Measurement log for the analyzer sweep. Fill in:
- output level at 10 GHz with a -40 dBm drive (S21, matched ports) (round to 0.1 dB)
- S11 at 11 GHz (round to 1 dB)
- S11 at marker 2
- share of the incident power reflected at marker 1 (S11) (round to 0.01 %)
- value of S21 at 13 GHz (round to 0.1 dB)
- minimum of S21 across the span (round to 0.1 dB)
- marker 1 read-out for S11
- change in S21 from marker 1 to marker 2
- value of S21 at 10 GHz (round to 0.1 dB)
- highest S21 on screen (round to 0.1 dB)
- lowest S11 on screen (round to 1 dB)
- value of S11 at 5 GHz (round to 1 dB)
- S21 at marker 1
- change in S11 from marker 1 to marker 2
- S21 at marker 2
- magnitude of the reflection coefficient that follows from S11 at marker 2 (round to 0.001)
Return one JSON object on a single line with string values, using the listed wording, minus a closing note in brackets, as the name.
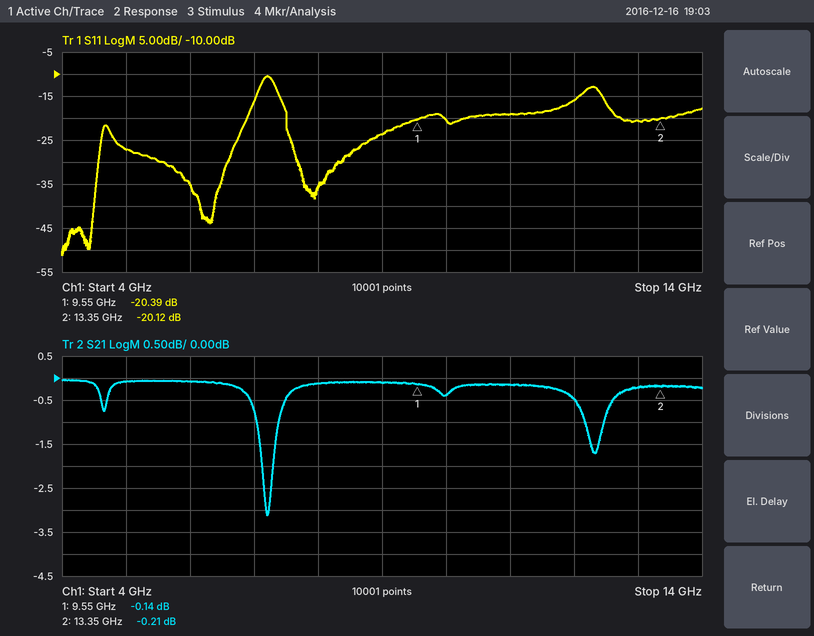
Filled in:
{"output level at 10 GHz with a -40 dBm drive (S21, matched ports)": "-40.4 dBm", "S11 at 11 GHz": "-19 dB", "S11 at marker 2": "-20.12 dB", "share of the incident power reflected at marker 1 (S11)": "0.91 %", "value of S21 at 13 GHz": "-0.2 dB", "minimum of S21 across the span": "-3.1 dB", "marker 1 read-out for S11": "-20.39 dB", "change in S21 from marker 1 to marker 2": "-0.07 dB", "value of S21 at 10 GHz": "-0.4 dB", "highest S21 on screen": "0.0 dB", "lowest S11 on screen": "-51 dB", "value of S11 at 5 GHz": "-27 dB", "S21 at marker 1": "-0.14 dB", "change in S11 from marker 1 to marker 2": "0.27 dB", "S21 at marker 2": "-0.21 dB", "magnitude of the reflection coefficient that follows from S11 at marker 2": "0.099"}
